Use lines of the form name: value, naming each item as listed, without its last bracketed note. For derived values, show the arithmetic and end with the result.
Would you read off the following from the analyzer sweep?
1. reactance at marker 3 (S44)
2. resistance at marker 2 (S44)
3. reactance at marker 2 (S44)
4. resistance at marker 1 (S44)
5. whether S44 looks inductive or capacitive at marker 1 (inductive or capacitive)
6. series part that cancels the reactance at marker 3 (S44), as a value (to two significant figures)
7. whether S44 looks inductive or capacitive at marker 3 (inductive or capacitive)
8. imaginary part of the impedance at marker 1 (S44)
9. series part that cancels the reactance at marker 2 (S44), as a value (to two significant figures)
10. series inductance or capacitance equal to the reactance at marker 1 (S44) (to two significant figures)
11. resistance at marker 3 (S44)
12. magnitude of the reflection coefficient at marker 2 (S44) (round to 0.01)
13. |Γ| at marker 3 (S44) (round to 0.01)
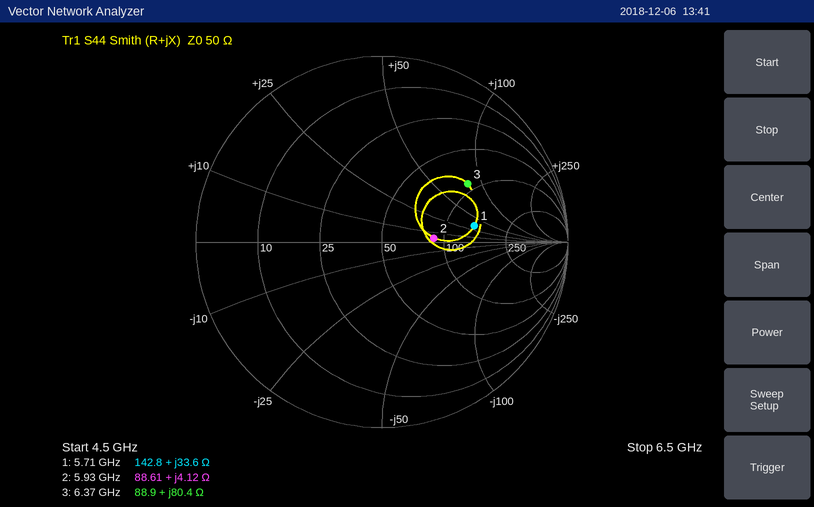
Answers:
reactance at marker 3: +80.4 Ω
resistance at marker 2: 88.61 Ω
reactance at marker 2: +4.12 Ω
resistance at marker 1: 142.8 Ω
whether S44 looks inductive or capacitive at marker 1: inductive
series part that cancels the reactance at marker 3 (S44), as a value: C = 1/(2π × 6.37 GHz × 80.4 Ω) ≈ 311 fF, so 310 fF to two significant figures
whether S44 looks inductive or capacitive at marker 3: inductive
imaginary part of the impedance at marker 1: +33.6 Ω
series part that cancels the reactance at marker 2 (S44), as a value: C = 1/(2π × 5.93 GHz × 4.12 Ω) ≈ 6.5 pF
series inductance or capacitance equal to the reactance at marker 1 (S44): L = 33.6 Ω/(2π × 5.71 GHz) ≈ 937 pH, so 940 pH to two significant figures
resistance at marker 3: 88.9 Ω
magnitude of the reflection coefficient at marker 2 (S44): 0.28
|Γ| at marker 3 (S44): 0.56
